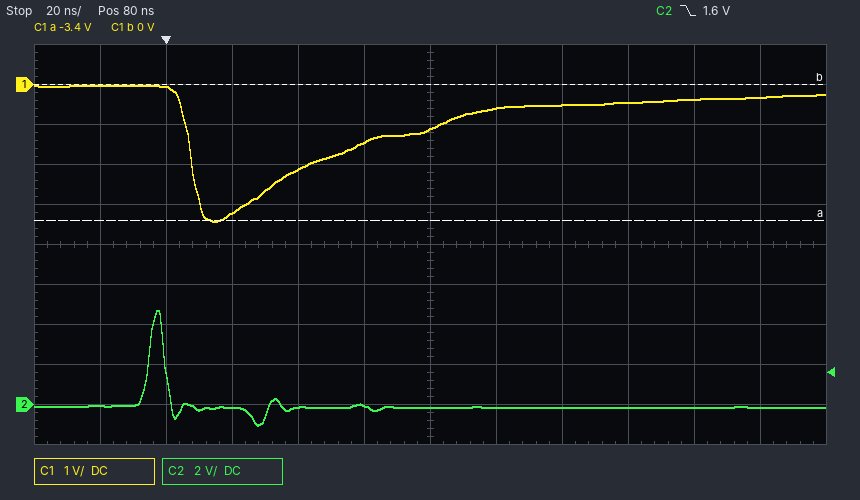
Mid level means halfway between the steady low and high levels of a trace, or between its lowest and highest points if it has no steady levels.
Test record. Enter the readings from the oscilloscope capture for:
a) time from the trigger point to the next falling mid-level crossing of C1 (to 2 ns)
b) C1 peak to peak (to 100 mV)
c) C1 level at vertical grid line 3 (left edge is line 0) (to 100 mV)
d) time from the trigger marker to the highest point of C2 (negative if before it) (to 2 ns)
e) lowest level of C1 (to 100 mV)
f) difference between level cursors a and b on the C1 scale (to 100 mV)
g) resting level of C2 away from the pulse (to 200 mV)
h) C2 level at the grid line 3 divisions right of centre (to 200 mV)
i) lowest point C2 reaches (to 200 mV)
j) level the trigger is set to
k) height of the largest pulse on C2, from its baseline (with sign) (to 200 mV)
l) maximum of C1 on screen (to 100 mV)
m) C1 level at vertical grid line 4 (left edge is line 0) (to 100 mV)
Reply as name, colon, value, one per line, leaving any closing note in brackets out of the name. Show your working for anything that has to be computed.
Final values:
time from the trigger point to the next falling mid-level crossing of C1: 8 ns
C1 peak to peak: 0.0 V − (-3.4 V) = 3.4 V
C1 level at vertical grid line 3 (left edge is line 0): -3.2 V
time from the trigger marker to the highest point of C2 (negative if before it): -2 ns
lowest level of C1: -3.4 V
difference between level cursors a and b on the C1 scale: 3.4 V
resting level of C2 away from the pulse: -200 mV
C2 level at the grid line 3 divisions right of centre: -200 mV
lowest point C2 reaches: -1.0 V
level the trigger is set to: 1.6 V
height of the largest pulse on C2, from its baseline (with sign): +4.8 V
maximum of C1 on screen: 0.0 V
C1 level at vertical grid line 4 (left edge is line 0): -2.1 V
